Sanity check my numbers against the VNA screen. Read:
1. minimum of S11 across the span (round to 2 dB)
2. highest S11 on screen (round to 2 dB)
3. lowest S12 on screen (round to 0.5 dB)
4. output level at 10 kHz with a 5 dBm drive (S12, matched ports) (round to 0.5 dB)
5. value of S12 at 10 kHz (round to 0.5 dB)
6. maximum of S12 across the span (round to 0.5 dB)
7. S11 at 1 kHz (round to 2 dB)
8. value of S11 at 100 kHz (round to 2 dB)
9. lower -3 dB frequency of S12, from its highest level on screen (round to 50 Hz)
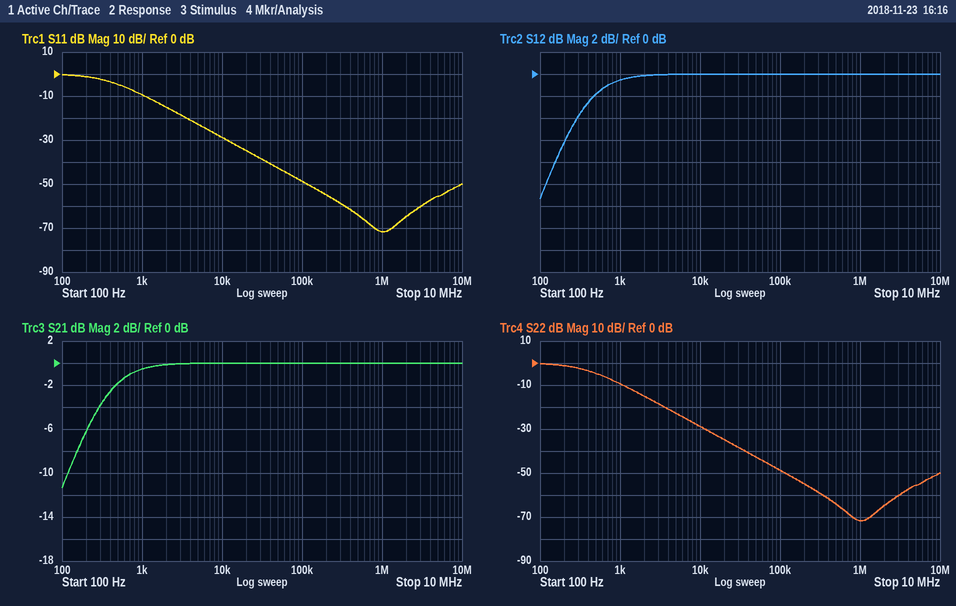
-72 dB
0 dB
-11.5 dB
5.0 dBm
0.0 dB
0.0 dB
-10 dB
-48 dB
350 Hz
